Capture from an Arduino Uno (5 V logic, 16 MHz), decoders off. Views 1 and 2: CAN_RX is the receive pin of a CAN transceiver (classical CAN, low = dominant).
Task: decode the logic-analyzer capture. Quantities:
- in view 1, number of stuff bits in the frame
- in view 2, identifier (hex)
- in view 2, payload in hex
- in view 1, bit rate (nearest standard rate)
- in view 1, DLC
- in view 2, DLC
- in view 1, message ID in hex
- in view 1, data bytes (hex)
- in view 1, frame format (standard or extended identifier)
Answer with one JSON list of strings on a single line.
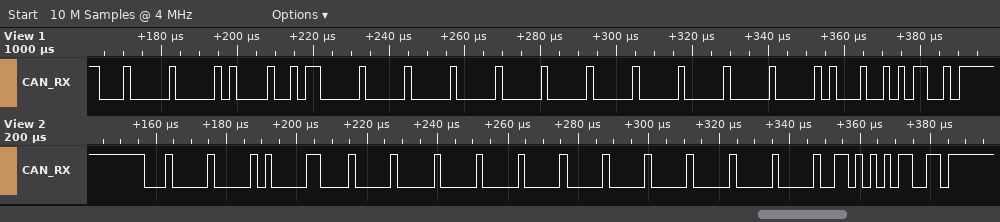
["13", "0x100", "21 00 00 00 00 00 00 00", "500 kbit/s", "8", "8", "0x100", "4B 00 00 00 00 00 00 00", "standard"]
